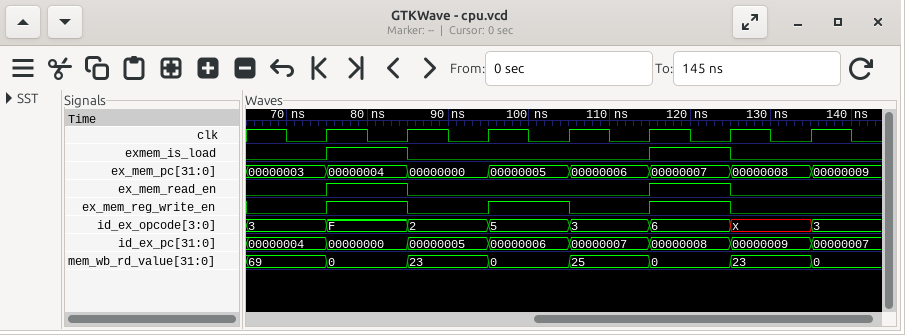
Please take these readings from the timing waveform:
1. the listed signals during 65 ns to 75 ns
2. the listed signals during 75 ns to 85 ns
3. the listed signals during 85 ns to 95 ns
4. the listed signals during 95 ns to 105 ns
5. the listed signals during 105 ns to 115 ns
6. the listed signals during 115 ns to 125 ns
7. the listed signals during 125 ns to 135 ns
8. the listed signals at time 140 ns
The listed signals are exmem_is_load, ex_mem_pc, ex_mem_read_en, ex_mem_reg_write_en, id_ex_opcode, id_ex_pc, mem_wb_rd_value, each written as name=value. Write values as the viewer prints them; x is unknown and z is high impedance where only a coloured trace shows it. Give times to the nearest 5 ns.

exmem_is_load=0, ex_mem_pc=00000003, ex_mem_read_en=0, ex_mem_reg_write_en=0, id_ex_opcode=3, id_ex_pc=00000004, mem_wb_rd_value=69
exmem_is_load=1, ex_mem_pc=00000004, ex_mem_read_en=1, ex_mem_reg_write_en=1, id_ex_opcode=F, id_ex_pc=00000000, mem_wb_rd_value=0
exmem_is_load=0, ex_mem_pc=00000000, ex_mem_read_en=0, ex_mem_reg_write_en=0, id_ex_opcode=2, id_ex_pc=00000005, mem_wb_rd_value=23
exmem_is_load=0, ex_mem_pc=00000005, ex_mem_read_en=0, ex_mem_reg_write_en=1, id_ex_opcode=5, id_ex_pc=00000006, mem_wb_rd_value=0
exmem_is_load=0, ex_mem_pc=00000006, ex_mem_read_en=0, ex_mem_reg_write_en=0, id_ex_opcode=3, id_ex_pc=00000007, mem_wb_rd_value=25
exmem_is_load=1, ex_mem_pc=00000007, ex_mem_read_en=1, ex_mem_reg_write_en=1, id_ex_opcode=6, id_ex_pc=00000008, mem_wb_rd_value=0
exmem_is_load=0, ex_mem_pc=00000008, ex_mem_read_en=0, ex_mem_reg_write_en=0, id_ex_opcode=x, id_ex_pc=00000009, mem_wb_rd_value=23
exmem_is_load=0, ex_mem_pc=00000009, ex_mem_read_en=0, ex_mem_reg_write_en=0, id_ex_opcode=3, id_ex_pc=00000007, mem_wb_rd_value=0
